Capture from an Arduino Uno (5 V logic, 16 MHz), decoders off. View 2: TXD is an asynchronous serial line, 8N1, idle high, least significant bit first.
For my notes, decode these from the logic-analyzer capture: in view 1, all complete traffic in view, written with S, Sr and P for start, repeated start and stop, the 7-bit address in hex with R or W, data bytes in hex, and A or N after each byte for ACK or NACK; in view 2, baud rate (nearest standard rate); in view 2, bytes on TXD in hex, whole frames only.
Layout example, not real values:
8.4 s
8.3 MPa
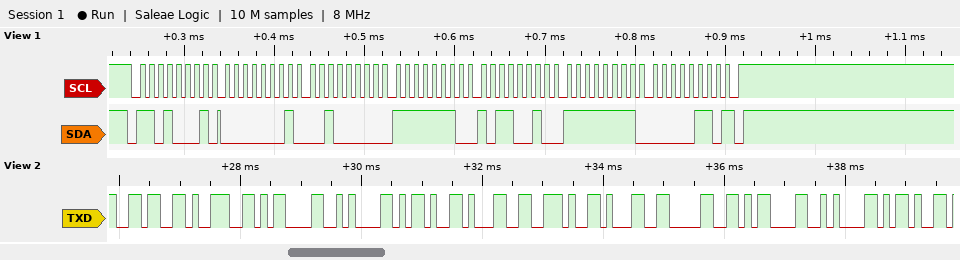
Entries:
S 68R A 01 A 20 A FE A B2 A FF A 06 N P
9600 baud
36 39 0D 0A 2D 31 2E 31 30 0D 0A 2D
